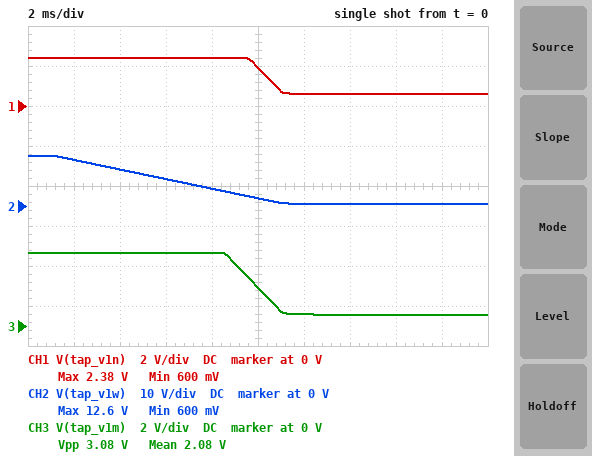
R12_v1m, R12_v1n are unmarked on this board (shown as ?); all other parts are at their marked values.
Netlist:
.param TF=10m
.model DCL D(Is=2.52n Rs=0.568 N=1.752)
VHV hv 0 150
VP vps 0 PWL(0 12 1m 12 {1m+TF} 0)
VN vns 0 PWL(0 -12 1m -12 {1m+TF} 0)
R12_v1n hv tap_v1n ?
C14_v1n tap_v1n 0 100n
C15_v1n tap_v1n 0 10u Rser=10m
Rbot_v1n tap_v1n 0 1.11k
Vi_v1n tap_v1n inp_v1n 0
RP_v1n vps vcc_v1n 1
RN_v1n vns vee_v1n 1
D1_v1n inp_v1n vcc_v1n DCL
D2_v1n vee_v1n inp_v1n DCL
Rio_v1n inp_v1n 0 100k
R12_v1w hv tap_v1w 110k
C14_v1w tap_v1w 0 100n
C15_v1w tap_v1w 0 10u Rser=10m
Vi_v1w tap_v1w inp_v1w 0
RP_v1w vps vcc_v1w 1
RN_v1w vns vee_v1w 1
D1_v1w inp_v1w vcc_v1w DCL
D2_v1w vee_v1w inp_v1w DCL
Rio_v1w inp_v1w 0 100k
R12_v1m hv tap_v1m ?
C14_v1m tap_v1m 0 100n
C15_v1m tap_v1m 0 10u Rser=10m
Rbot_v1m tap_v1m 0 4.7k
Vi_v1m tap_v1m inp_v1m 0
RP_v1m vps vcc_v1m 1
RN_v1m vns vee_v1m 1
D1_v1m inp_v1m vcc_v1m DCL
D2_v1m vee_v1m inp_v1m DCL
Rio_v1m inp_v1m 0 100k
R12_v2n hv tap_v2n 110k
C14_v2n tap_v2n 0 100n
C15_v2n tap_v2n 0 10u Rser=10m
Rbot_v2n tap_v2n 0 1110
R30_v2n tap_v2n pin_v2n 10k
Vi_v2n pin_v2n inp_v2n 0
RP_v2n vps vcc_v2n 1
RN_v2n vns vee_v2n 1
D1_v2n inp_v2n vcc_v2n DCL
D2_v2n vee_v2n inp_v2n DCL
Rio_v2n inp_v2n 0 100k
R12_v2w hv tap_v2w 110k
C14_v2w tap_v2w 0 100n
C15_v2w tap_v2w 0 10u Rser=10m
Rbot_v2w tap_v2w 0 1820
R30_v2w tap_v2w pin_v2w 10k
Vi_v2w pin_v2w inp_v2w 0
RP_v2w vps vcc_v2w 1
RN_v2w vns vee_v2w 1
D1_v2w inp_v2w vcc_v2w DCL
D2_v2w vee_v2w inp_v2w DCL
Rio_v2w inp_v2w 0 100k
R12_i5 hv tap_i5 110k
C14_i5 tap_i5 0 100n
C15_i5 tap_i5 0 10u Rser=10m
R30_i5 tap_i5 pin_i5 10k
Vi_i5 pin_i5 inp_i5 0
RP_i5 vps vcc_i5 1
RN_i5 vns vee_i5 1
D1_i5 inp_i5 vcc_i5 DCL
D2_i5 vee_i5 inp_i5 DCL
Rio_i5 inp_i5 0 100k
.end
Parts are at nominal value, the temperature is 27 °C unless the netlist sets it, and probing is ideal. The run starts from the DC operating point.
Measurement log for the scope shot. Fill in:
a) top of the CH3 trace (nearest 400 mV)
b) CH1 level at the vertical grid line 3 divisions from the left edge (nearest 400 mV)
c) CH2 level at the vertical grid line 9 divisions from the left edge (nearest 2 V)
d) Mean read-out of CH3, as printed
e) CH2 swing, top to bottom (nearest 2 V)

3.6 V
2.4 V
0 V
2.08 V
12 V
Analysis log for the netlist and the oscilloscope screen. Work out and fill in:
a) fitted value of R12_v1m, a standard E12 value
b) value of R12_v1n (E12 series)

180 kΩ
68 kΩ
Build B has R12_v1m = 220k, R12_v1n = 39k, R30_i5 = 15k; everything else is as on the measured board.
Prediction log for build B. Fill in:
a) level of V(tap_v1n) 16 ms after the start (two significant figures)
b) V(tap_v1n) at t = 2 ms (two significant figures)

640 mV
4.1 V
